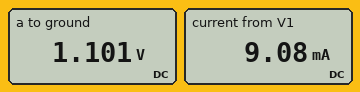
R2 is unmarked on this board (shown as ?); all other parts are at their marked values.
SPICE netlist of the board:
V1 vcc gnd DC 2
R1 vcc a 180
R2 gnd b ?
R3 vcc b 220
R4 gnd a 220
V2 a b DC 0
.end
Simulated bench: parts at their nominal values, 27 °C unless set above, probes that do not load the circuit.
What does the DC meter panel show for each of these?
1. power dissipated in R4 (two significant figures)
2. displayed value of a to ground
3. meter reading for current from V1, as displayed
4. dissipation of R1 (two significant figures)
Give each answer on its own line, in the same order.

5.5 mW
1.101 V
9.08 mA
4.5 mW
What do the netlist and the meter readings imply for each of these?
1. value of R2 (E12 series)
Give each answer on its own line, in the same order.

270 Ω
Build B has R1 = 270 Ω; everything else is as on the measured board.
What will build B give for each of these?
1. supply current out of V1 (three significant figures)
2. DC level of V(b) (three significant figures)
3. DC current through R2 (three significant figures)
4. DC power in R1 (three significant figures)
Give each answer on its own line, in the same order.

8.25 mA
1.00 V
3.70 mA
3.70 mW
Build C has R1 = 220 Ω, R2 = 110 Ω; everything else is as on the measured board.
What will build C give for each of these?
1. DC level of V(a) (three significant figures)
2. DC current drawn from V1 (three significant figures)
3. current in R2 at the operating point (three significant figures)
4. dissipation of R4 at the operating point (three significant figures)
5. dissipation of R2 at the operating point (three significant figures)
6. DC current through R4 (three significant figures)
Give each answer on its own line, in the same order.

800 mV
10.9 mA
7.27 mA
2.91 mW
5.82 mW
3.64 mA
